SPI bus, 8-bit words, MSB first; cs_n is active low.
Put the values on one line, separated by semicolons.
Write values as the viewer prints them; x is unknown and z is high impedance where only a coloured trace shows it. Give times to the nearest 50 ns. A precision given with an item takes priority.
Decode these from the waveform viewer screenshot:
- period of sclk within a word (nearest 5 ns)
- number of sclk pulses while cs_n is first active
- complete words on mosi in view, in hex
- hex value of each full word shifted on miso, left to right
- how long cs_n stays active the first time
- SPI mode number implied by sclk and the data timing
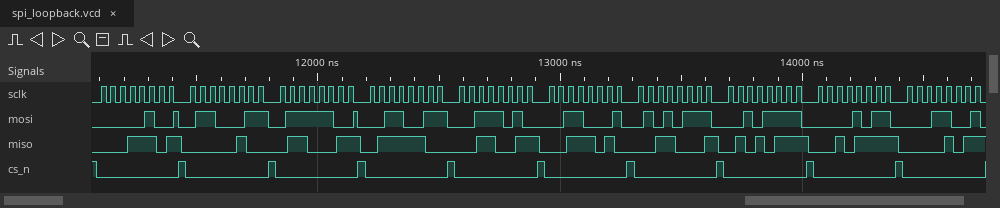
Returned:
40 ns; 8; 04, 63, 7C, 33, 3A, 31, 57, 2F, 0B, 19; 1D, 04, 63, 7C, 33, 3A, 31, 57, 2F, 0B; 350 ns; 0
